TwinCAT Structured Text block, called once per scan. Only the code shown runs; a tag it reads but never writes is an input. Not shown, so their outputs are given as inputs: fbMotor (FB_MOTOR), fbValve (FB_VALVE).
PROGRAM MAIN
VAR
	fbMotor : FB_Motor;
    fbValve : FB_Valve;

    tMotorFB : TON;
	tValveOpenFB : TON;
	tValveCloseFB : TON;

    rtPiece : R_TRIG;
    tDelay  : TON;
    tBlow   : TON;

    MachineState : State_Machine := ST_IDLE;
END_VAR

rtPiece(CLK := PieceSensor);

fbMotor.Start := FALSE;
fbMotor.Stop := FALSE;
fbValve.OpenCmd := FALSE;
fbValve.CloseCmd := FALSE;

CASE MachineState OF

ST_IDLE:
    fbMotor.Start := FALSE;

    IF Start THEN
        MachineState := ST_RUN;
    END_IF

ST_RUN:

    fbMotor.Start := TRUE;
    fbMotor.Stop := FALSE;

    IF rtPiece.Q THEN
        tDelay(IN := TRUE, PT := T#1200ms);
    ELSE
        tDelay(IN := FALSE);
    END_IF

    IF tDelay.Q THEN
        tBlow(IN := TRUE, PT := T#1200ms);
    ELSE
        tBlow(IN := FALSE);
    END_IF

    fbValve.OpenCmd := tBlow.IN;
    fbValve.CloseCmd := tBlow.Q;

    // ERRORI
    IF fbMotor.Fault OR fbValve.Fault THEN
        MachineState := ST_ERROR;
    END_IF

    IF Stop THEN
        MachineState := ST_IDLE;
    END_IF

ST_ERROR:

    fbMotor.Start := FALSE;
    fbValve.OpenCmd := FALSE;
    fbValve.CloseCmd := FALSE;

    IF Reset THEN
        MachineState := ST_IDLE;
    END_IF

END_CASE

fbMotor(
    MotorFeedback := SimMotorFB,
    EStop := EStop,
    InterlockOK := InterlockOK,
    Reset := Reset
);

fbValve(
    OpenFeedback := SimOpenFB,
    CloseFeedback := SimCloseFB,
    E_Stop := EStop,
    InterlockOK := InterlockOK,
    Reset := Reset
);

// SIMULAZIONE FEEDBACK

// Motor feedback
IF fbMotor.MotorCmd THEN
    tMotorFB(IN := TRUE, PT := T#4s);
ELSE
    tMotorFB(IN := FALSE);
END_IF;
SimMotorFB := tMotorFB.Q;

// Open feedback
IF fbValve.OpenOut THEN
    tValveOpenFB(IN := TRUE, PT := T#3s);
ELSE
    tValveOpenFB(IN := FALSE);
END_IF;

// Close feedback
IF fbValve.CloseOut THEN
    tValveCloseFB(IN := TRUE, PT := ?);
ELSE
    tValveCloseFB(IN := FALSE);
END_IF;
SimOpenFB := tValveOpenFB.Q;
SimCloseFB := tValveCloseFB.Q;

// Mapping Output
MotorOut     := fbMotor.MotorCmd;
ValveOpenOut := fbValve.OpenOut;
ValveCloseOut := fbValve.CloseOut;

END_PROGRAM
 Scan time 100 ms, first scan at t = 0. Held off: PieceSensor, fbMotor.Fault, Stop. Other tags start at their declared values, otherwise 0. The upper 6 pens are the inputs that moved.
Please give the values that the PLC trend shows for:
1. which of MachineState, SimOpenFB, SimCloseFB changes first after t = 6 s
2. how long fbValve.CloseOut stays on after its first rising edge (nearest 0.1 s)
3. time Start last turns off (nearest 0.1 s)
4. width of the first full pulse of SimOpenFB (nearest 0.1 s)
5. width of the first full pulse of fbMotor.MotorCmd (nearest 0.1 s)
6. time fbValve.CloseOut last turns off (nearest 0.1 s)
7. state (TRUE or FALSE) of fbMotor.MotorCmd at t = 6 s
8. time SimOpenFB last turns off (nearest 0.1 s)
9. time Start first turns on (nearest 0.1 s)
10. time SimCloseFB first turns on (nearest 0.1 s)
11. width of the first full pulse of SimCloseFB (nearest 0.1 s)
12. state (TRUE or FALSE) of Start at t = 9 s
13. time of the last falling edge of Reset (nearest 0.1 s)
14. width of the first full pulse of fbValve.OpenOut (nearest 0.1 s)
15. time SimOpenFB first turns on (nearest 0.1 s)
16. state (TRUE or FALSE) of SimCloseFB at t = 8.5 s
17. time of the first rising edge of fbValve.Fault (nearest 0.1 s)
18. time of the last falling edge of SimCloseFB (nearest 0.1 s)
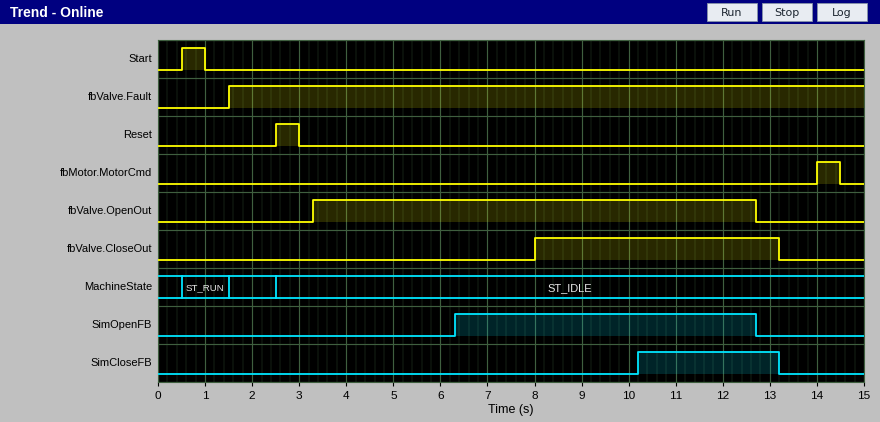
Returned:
SimOpenFB
5.2 s
1.0 s
6.4 s
0.5 s
13.2 s
FALSE
12.7 s
0.5 s
10.2 s
3.0 s
FALSE
3.0 s
9.4 s
6.3 s
FALSE
1.5 s
13.2 s
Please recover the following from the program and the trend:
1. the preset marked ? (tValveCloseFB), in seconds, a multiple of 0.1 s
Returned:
2.2 s
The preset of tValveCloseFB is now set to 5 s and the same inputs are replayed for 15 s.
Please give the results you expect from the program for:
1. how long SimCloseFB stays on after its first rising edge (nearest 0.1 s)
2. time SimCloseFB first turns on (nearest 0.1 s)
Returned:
0.2 s
13.0 s
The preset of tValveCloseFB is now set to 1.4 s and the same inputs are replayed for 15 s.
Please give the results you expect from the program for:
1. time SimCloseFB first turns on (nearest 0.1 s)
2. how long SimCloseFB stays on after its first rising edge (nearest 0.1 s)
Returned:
9.4 s
3.8 s
